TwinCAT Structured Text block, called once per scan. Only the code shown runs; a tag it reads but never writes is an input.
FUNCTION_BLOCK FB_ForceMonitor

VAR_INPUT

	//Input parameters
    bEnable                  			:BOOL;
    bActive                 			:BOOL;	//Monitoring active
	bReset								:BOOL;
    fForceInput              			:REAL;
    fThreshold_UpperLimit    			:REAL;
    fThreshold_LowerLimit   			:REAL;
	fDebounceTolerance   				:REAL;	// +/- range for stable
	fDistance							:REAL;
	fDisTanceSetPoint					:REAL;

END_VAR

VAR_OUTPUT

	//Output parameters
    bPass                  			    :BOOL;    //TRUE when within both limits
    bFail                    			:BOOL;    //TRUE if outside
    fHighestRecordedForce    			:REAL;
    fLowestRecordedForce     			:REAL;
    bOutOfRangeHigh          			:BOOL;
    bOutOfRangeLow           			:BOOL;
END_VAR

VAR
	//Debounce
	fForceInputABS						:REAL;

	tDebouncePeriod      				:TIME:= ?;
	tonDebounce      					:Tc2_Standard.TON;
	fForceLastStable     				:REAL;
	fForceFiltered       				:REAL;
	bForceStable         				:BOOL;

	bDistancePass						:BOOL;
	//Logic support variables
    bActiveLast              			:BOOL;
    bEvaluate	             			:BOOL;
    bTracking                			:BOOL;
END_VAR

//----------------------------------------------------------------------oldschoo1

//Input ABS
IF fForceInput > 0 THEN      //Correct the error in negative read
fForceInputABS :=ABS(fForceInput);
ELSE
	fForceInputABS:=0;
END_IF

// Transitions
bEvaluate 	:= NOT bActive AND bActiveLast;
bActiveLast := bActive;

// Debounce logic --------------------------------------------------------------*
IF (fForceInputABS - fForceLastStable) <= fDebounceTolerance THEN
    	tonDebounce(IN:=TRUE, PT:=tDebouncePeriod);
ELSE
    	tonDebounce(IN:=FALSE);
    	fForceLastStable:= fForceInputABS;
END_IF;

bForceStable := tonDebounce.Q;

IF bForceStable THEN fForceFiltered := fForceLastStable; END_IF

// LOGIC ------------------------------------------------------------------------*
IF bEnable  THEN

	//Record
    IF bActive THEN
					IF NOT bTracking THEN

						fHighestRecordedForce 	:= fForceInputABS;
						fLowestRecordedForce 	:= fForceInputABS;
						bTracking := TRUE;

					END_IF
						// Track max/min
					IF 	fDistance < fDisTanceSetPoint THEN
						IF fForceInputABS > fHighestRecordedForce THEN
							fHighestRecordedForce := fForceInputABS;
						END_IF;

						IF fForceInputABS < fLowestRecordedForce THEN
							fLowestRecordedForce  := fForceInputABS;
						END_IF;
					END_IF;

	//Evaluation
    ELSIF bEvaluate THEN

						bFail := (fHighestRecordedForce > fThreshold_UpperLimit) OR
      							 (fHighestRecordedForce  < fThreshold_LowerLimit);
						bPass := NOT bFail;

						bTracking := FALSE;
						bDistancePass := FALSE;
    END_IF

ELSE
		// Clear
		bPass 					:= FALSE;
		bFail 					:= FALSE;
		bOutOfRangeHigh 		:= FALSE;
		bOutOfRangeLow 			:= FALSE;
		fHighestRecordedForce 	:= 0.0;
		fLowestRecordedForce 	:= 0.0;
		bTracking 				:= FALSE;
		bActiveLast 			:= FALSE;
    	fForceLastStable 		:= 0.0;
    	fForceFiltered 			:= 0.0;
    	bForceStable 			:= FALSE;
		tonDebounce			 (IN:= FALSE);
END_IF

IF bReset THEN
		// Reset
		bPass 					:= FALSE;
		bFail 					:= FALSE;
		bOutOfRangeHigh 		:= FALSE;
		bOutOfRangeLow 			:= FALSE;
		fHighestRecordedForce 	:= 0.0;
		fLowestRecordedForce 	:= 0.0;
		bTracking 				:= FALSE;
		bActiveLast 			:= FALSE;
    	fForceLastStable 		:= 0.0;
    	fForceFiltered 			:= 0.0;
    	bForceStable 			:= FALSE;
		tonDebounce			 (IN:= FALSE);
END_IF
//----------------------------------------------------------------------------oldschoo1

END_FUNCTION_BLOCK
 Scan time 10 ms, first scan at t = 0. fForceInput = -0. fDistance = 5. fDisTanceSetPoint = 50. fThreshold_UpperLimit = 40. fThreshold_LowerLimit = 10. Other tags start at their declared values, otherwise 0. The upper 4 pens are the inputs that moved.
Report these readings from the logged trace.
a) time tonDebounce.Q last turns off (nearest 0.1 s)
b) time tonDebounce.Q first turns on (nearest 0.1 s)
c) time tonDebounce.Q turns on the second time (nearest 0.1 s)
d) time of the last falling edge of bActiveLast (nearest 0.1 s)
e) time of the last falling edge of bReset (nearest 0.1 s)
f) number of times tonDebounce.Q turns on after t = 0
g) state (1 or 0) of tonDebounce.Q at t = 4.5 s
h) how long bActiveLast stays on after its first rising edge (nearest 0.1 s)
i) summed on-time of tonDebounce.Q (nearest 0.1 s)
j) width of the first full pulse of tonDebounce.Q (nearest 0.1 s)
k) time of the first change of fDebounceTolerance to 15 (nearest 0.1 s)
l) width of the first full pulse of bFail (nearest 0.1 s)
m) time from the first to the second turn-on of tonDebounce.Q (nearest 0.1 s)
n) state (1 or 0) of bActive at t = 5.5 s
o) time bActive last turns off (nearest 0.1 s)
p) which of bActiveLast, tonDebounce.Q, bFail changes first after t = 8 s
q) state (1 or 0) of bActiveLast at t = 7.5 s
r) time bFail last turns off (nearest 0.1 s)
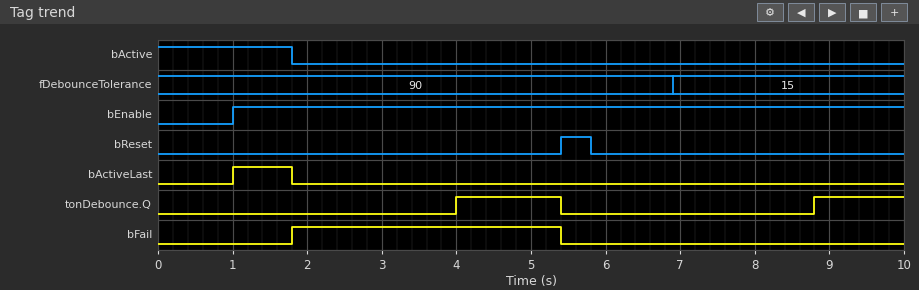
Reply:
5.4 s
4.0 s
8.8 s
1.8 s
5.8 s
2
1
0.8 s
2.6 s
1.4 s
6.9 s
3.6 s
4.8 s
0
1.8 s
tonDebounce.Q
0
5.4 s
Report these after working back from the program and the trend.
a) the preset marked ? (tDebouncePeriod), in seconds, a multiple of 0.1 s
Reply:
3.0 s
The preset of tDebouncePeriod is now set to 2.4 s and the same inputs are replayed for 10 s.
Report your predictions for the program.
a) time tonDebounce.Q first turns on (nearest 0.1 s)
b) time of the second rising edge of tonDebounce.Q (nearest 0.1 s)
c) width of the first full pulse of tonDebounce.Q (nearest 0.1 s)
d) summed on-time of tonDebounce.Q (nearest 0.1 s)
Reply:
3.4 s
8.2 s
2.0 s
3.8 s
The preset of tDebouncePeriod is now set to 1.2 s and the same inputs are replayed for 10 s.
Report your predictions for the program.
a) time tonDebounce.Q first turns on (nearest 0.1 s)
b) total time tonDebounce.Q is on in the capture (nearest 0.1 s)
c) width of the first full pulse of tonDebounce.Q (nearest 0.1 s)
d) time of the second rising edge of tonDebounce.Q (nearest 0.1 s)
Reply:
2.2 s
6.2 s
3.2 s
7.0 s
